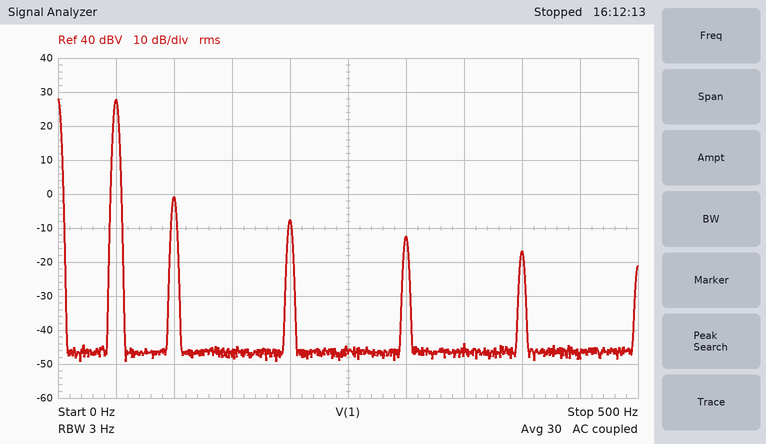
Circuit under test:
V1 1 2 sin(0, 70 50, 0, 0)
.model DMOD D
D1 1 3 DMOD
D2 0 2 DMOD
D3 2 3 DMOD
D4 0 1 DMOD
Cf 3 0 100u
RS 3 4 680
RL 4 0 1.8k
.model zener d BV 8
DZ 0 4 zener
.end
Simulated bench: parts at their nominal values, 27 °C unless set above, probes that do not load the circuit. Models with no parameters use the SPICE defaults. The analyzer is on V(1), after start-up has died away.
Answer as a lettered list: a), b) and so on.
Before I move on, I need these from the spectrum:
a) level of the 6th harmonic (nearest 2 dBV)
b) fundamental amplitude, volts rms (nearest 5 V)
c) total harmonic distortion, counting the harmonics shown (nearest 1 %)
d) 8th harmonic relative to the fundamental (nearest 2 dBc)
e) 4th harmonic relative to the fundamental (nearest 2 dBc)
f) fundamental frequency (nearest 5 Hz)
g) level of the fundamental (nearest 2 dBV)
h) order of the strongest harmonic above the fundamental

a) -12 dBV
b) 25 V
c) 4 %
d) -44 dBc
e) -36 dBc
f) 50 Hz
g) 28 dBV
h) 2
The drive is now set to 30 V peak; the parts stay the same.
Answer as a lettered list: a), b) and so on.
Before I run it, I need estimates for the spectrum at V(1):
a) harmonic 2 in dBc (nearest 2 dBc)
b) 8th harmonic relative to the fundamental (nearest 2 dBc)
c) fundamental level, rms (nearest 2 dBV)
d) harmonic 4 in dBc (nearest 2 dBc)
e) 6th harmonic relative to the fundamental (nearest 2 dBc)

a) -30 dBc
b) -46 dBc
c) 20 dBV
d) -38 dBc
e) -42 dBc
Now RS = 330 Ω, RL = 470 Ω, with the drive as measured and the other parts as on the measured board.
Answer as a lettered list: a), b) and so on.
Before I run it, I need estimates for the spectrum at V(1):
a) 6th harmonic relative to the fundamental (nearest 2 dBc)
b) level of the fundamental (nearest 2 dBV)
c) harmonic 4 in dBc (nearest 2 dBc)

a) -36 dBc
b) 28 dBV
c) -30 dBc
